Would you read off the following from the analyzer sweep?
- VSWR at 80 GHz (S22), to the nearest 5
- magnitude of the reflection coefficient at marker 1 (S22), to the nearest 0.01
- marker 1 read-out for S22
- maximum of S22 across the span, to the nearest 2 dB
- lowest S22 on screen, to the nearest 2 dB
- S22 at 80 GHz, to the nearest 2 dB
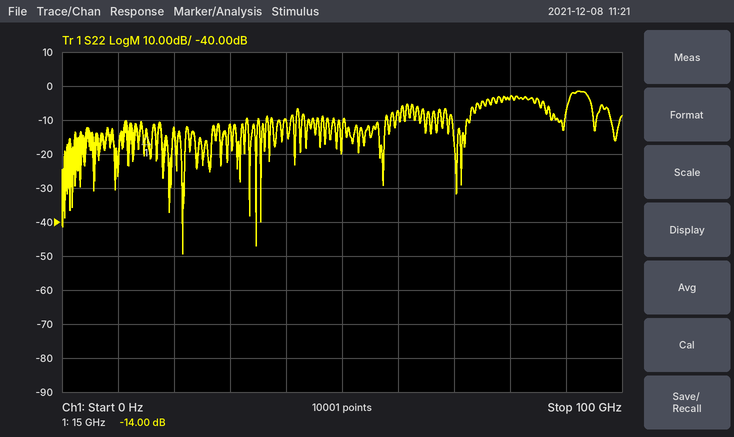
5
0.20
-14.00 dB
-2 dB
-50 dB
-4 dB
